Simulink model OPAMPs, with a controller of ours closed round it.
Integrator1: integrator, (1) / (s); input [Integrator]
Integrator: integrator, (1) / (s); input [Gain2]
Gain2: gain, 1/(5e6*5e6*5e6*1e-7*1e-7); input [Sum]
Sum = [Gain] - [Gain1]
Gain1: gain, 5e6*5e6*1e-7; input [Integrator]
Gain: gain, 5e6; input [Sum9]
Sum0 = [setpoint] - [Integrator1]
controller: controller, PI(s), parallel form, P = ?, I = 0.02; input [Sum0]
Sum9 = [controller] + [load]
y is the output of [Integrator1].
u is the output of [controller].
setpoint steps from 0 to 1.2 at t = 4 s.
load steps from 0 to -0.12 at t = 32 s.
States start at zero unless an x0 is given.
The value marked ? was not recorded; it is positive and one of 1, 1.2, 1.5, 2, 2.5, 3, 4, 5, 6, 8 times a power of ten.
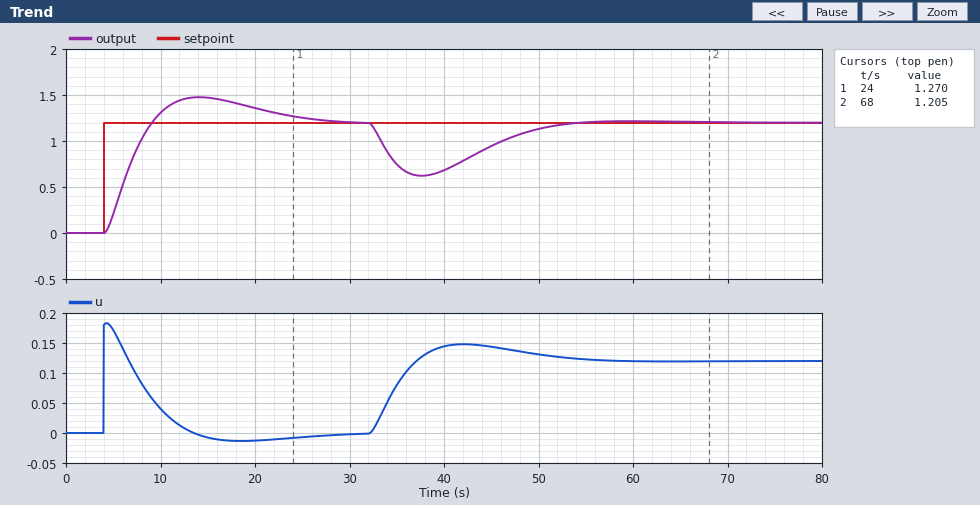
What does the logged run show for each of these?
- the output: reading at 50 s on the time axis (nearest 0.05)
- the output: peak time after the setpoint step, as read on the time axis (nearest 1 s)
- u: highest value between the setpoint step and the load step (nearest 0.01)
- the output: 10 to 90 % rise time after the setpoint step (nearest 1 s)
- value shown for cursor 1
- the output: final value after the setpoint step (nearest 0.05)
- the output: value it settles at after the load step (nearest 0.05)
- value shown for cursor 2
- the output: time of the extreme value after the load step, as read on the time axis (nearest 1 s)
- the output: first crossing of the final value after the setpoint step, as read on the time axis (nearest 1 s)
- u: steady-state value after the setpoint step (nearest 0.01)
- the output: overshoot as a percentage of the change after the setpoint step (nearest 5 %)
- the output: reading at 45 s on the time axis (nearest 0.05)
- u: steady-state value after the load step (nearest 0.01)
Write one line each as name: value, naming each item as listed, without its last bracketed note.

the output: reading at 50 s on the time axis: 1.15
the output: peak time after the setpoint step, as read on the time axis: 14 s
u: highest value between the setpoint step and the load step: 0.18
the output: 10 to 90 % rise time after the setpoint step: 4 s
value shown for cursor 1: 1.270
the output: final value after the setpoint step: 1.20
the output: value it settles at after the load step: 1.20
value shown for cursor 2: 1.205
the output: time of the extreme value after the load step, as read on the time axis: 38 s
the output: first crossing of the final value after the setpoint step, as read on the time axis: 9 s
u: steady-state value after the setpoint step: 0.00
the output: overshoot as a percentage of the change after the setpoint step: 25 %
the output: reading at 45 s on the time axis: 0.95
u: steady-state value after the load step: 0.12
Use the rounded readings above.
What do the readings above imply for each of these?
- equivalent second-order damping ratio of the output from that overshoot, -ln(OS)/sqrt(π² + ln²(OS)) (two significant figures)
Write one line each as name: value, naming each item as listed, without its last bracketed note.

equivalent second-order damping ratio of the output from that overshoot, -ln(OS)/sqrt(π² + ln²(OS)): 0.40
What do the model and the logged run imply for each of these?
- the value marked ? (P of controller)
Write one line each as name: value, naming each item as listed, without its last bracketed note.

the value marked ?: 0.15
